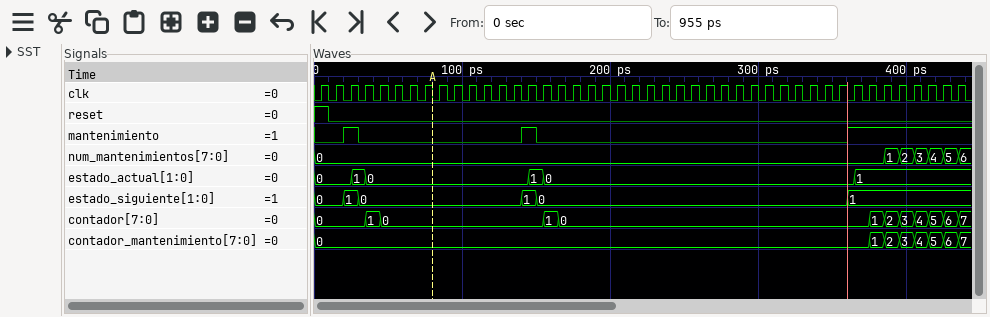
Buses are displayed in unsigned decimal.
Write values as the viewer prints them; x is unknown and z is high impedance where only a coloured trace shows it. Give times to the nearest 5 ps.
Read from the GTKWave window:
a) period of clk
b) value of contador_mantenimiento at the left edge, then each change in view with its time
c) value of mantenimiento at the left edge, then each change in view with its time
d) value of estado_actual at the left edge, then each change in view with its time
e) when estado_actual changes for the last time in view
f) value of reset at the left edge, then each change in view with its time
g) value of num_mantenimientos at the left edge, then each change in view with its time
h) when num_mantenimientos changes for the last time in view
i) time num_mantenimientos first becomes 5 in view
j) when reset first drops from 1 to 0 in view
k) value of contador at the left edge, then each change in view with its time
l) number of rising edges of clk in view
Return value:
10 ps
0, 1 at 375 ps, 2 at 385 ps, 3 at 395 ps, 4 at 405 ps, 5 at 415 ps, 6 at 425 ps, 7 at 435 ps
0, 1 at 20 ps, 0 at 30 ps, 1 at 140 ps, 0 at 150 ps, 1 at 360 ps
0, 1 at 25 ps, 0 at 35 ps, 1 at 145 ps, 0 at 155 ps, 1 at 365 ps
365 ps
1, 0 at 10 ps
0, 1 at 385 ps, 2 at 395 ps, 3 at 405 ps, 4 at 415 ps, 5 at 425 ps, 6 at 435 ps
435 ps
425 ps
10 ps
0, 1 at 35 ps, 0 at 45 ps, 1 at 155 ps, 0 at 165 ps, 1 at 375 ps, 2 at 385 ps, 3 at 395 ps, 4 at 405 ps, 5 at 415 ps, 6 at 425 ps, 7 at 435 ps
44
